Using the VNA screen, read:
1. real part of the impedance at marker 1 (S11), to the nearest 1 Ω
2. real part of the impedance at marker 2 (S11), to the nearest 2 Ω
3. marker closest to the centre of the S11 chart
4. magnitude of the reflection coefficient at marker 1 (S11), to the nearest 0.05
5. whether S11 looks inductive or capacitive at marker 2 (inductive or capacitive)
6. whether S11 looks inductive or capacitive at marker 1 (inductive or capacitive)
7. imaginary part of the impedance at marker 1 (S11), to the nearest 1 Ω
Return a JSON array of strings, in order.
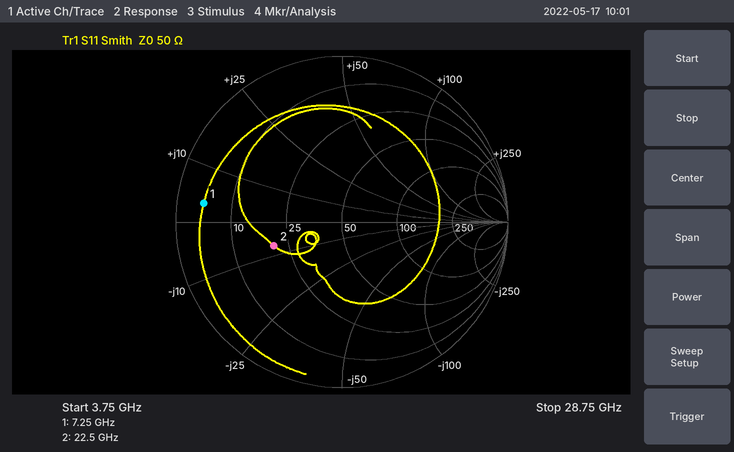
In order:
["4 Ω", "20 Ω", "marker 2", "0.85", "capacitive", "inductive", "+3 Ω"]
